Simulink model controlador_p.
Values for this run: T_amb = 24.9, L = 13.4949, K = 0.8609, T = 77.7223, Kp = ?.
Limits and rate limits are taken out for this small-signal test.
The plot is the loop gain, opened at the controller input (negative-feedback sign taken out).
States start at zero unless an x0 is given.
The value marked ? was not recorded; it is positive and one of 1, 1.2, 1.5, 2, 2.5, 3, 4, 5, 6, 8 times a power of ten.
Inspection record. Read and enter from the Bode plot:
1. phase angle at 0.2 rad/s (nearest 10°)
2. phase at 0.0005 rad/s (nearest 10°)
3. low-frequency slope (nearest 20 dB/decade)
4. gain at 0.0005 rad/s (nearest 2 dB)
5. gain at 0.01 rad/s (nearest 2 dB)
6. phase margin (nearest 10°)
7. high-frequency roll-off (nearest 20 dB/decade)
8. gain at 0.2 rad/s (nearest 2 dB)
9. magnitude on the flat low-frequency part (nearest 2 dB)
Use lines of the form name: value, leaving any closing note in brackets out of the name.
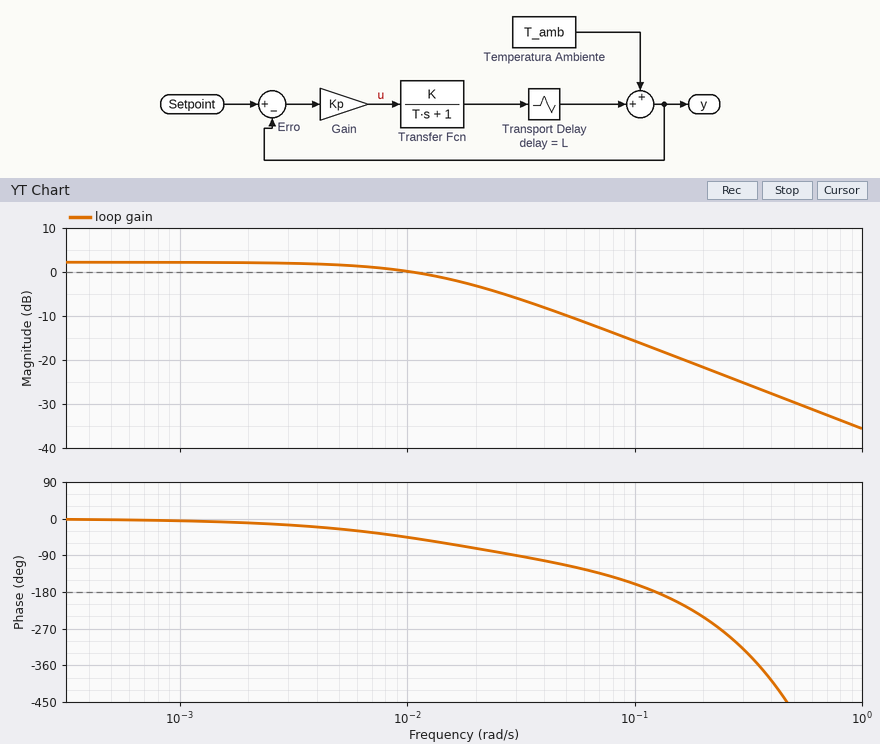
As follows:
phase angle at 0.2 rad/s: -240°
phase at 0.0005 rad/s: 0°
low-frequency slope: 0 dB/decade
gain at 0.0005 rad/s: 2 dB
gain at 0.01 rad/s: 0 dB
phase margin: 130°
high-frequency roll-off: -20 dB/decade
gain at 0.2 rad/s: -22 dB
magnitude on the flat low-frequency part: 2 dB
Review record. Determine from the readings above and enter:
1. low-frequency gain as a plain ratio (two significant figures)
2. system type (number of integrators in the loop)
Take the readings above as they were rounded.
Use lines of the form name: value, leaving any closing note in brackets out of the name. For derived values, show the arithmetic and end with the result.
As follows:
low-frequency gain as a plain ratio: 10^(2 / 20) = 1.3
system type: 0
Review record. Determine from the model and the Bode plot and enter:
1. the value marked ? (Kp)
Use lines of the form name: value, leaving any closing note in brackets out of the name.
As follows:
the value marked ?: 1.5
